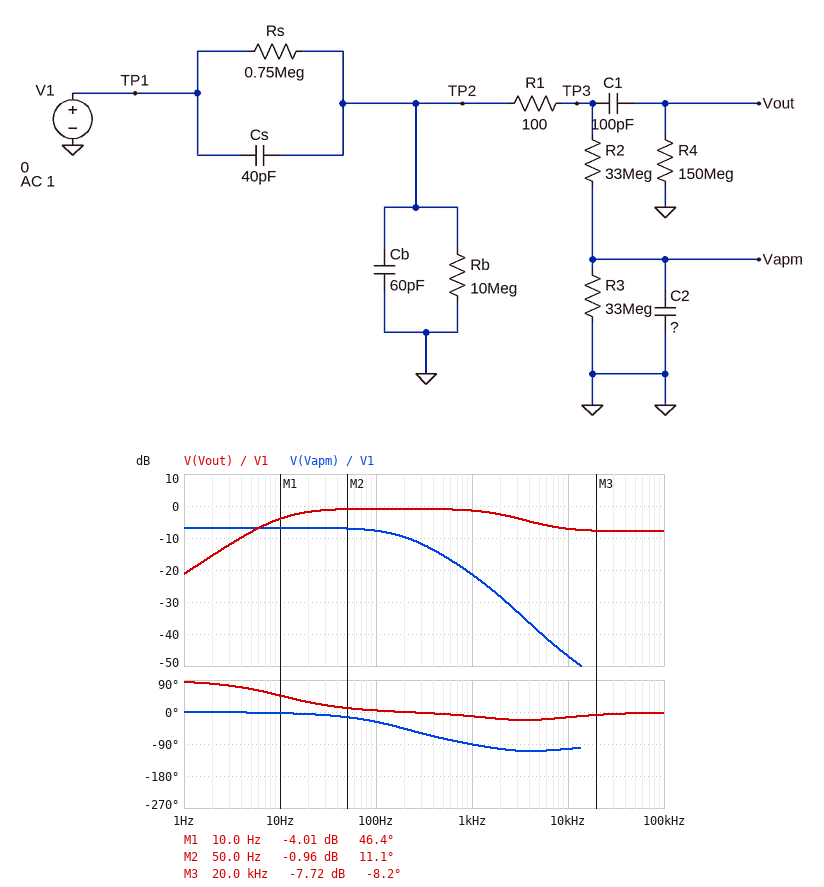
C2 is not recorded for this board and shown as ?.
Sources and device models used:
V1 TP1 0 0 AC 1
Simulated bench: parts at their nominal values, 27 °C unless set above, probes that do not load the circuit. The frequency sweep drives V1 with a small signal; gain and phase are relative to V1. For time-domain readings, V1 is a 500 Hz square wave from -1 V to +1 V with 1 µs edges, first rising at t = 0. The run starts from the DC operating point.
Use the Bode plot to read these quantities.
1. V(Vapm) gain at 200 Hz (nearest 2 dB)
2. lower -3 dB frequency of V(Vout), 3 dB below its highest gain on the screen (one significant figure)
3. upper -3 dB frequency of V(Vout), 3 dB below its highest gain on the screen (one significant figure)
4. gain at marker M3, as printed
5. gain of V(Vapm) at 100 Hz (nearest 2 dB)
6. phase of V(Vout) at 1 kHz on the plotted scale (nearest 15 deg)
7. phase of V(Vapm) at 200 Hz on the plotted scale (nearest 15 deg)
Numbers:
-10 dB
10 Hz
3 kHz
-7.72 dB
-8 dB
-15 deg
-45 deg
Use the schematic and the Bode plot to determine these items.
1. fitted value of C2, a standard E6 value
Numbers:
47 pF
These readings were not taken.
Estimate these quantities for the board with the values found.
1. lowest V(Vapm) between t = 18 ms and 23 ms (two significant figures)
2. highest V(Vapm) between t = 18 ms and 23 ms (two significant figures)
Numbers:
-250 mV
250 mV
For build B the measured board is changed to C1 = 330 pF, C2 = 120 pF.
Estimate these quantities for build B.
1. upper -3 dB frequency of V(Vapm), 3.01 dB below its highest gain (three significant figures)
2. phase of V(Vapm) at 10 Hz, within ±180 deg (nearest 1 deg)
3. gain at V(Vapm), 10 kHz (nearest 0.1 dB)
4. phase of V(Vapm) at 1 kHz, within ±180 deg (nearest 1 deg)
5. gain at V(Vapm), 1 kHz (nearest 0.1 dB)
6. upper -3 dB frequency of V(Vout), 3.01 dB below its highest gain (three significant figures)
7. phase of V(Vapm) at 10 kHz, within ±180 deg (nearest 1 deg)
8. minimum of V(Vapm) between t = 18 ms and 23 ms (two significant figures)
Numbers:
78.7 Hz
-7 deg
-55.0 dB
-98 deg
-29.4 dB
2.95 kHz
-104 deg
-110 mV
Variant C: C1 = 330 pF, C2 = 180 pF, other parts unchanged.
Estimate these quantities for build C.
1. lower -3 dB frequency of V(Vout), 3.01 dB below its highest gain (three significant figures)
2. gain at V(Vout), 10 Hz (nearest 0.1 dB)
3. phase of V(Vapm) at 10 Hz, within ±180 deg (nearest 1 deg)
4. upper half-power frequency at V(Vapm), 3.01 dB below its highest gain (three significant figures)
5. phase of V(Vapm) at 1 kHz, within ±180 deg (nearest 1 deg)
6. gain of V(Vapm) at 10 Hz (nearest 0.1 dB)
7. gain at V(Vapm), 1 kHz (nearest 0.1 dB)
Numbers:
3.16 Hz
-1.2 dB
-11 deg
52.5 Hz
-99 deg
-6.9 dB
-32.9 dB
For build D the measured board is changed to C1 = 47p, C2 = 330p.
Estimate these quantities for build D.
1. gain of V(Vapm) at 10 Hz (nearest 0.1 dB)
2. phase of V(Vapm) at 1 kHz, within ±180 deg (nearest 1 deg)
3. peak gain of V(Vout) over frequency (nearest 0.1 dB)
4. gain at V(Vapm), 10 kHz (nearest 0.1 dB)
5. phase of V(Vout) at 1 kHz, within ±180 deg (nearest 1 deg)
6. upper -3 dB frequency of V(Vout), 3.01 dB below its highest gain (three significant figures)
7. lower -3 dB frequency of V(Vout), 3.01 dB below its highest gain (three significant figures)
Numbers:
-7.2 dB
-101 deg
-0.9 dB
-63.8 dB
-11 deg
3.06 kHz
21.8 Hz
